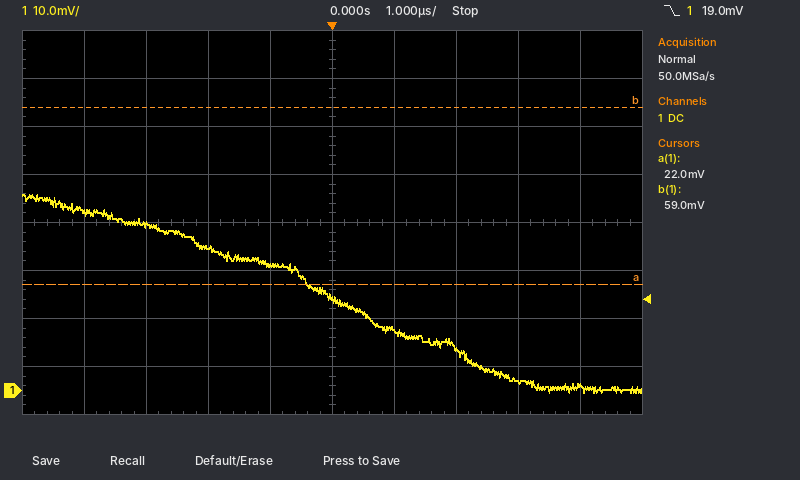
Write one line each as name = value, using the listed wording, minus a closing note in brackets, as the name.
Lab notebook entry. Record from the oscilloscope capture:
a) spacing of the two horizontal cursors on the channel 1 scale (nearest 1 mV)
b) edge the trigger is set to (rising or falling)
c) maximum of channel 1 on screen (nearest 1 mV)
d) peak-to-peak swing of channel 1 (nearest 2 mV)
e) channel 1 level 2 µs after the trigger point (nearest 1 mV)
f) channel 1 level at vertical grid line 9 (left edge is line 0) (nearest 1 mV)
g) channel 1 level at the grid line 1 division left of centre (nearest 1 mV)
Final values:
spacing of the two horizontal cursors on the channel 1 scale = 37 mV
edge the trigger is set to = falling
maximum of channel 1 on screen = 41 mV
peak-to-peak swing of channel 1 = 42 mV
channel 1 level 2 µs after the trigger point = 9 mV
channel 1 level at vertical grid line 9 (left edge is line 0) = 1 mV
channel 1 level at the grid line 1 division left of centre = 26 mV
